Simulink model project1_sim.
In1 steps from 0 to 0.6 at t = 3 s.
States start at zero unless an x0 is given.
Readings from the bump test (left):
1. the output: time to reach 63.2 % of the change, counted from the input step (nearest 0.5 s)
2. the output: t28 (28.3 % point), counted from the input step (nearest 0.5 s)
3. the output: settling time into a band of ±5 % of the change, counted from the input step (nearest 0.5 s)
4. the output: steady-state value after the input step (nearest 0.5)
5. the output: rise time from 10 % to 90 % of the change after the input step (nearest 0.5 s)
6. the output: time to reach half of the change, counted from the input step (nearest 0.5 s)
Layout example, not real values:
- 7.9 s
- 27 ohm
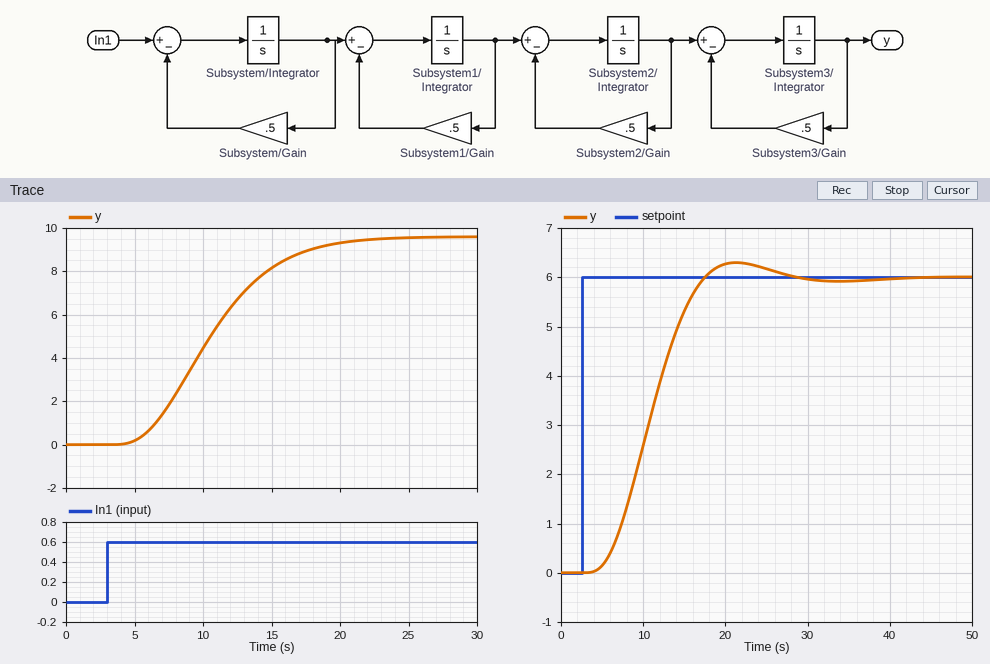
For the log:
- 8.5 s
- 5.5 s
- 15.5 s
- 9.5
- 10.0 s
- 7.5 s
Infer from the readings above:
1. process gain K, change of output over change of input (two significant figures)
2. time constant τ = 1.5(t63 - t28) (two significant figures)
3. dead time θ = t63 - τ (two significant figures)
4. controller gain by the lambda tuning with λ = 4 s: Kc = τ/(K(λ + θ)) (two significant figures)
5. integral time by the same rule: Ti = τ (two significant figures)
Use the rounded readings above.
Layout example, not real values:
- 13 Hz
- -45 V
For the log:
- 16
- 4.5 s
- 4.0 s
- 0.035
- 4.5 s
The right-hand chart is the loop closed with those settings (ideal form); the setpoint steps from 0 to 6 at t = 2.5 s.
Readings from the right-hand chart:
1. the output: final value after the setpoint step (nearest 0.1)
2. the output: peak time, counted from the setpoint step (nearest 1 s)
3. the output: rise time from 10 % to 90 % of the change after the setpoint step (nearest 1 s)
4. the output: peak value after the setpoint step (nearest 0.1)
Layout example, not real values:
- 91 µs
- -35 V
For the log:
- 6.0
- 19 s
- 9 s
- 6.3
